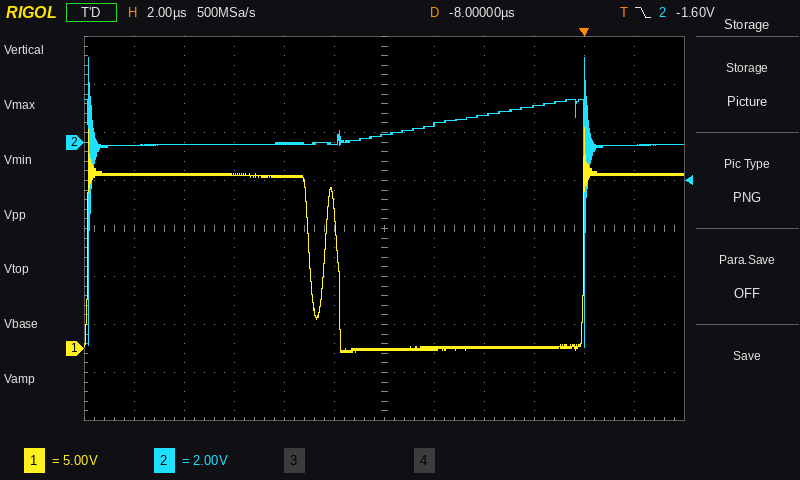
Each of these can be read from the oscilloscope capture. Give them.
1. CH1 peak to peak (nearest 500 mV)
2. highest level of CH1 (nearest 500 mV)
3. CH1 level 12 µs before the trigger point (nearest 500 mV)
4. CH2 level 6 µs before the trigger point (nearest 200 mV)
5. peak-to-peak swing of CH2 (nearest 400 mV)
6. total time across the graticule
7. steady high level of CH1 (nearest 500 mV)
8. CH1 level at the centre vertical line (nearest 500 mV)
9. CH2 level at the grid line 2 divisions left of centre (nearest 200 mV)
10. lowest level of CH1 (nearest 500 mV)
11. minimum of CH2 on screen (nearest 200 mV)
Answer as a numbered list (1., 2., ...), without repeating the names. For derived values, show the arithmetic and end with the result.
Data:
1. 23.0 V − (-500 mV) = 23.5 V
2. 23.0 V
3. 18.0 V
4. 800 mV
5. 12.0 V
6. 24 µs
7. 18.0 V
8. 0.0 V
9. 0.0 V
10. -500 mV
11. -8.6 V
